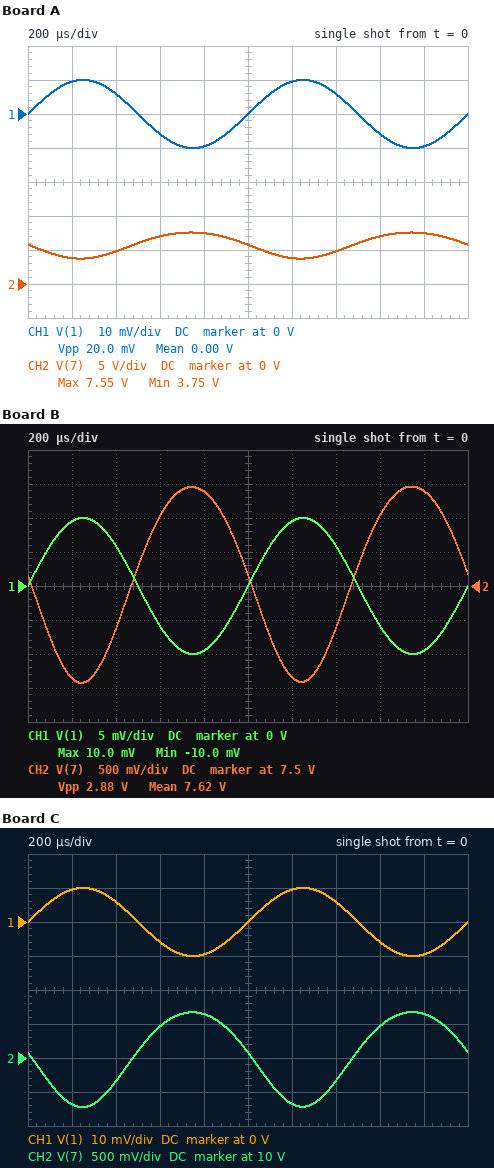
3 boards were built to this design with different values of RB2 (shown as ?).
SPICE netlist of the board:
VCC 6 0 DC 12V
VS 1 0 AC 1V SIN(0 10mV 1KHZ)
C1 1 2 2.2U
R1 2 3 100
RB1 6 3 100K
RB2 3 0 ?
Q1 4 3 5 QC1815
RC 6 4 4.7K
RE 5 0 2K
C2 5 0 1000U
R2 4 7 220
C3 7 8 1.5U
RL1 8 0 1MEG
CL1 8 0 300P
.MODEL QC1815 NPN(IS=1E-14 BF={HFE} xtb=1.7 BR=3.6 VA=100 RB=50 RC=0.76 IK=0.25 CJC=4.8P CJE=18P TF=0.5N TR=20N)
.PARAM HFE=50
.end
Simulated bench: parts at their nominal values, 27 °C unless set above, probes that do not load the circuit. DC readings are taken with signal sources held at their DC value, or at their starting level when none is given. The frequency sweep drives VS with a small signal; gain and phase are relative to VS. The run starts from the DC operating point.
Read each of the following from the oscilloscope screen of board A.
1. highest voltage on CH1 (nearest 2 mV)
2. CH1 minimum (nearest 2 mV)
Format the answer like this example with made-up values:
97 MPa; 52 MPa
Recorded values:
10 mV; -10 mV
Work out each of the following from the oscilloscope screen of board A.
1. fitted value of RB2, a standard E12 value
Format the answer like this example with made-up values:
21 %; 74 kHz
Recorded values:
56 kΩ
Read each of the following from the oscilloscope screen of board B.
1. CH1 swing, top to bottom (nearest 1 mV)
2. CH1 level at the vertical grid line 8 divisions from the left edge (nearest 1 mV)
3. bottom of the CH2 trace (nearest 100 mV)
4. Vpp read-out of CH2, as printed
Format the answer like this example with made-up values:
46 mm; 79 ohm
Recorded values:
20 mV; -6 mV; 6.1 V; 2.88 V
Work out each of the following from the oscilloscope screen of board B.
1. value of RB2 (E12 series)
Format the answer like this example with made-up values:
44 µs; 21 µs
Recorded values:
33 kΩ
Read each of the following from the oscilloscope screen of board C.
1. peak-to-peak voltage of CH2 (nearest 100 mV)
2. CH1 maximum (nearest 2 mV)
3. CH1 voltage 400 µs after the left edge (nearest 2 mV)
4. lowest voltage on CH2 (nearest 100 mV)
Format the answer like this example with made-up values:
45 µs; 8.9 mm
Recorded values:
1.4 V; 10 mV; 6 mV; 9.3 V
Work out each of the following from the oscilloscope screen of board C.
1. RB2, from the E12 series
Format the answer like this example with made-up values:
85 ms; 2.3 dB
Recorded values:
15 kΩ
